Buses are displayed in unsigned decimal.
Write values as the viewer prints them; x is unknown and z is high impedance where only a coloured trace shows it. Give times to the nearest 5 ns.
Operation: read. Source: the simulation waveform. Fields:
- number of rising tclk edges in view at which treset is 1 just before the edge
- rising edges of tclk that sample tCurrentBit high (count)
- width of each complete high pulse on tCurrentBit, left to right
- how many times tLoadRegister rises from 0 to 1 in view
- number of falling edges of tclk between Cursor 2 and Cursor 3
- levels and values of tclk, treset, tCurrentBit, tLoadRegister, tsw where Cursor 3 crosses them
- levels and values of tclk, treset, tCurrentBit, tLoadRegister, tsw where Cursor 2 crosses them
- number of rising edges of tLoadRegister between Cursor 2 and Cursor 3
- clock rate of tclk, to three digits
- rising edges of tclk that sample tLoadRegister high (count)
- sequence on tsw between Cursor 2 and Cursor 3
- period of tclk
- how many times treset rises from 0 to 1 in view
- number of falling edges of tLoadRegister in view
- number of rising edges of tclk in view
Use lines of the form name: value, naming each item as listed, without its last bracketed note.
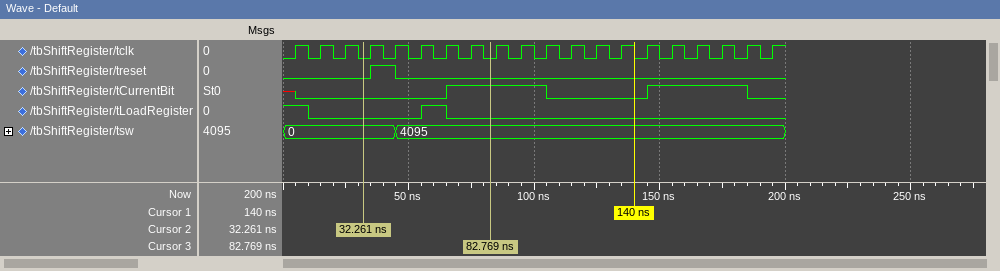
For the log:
number of rising tclk edges in view at which treset is 1 just before the edge: 1
rising edges of tclk that sample tCurrentBit high: 8
width of each complete high pulse on tCurrentBit, left to right: 40 ns, 40 ns
how many times tLoadRegister rises from 0 to 1 in view: 1
number of falling edges of tclk between Cursor 2 and Cursor 3: 5
levels and values of tclk, treset, tCurrentBit, tLoadRegister, tsw where Cursor 3 crosses them: tclk=0, treset=0, tCurrentBit=1, tLoadRegister=0, tsw=4095
levels and values of tclk, treset, tCurrentBit, tLoadRegister, tsw where Cursor 2 crosses them: tclk=0, treset=0, tCurrentBit=0, tLoadRegister=0, tsw=0
number of rising edges of tLoadRegister between Cursor 2 and Cursor 3: 1
clock rate of tclk, to three digits: 100 MHz
rising edges of tclk that sample tLoadRegister high: 2
sequence on tsw between Cursor 2 and Cursor 3: 0, 4095
period of tclk: 10 ns
how many times treset rises from 0 to 1 in view: 1
number of falling edges of tLoadRegister in view: 2
number of rising edges of tclk in view: 20
